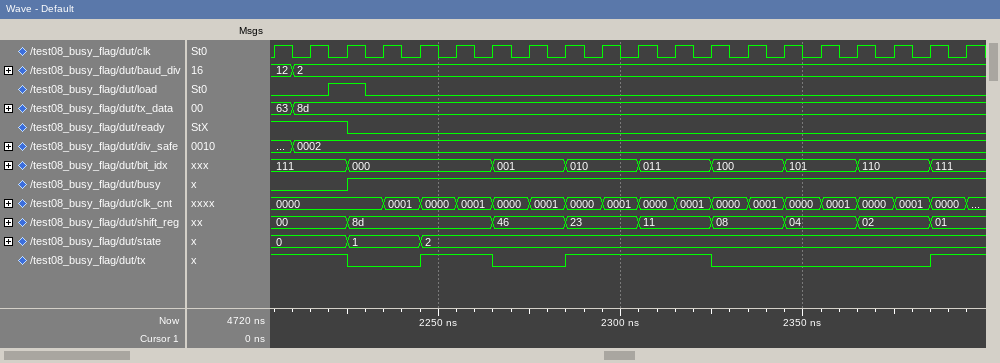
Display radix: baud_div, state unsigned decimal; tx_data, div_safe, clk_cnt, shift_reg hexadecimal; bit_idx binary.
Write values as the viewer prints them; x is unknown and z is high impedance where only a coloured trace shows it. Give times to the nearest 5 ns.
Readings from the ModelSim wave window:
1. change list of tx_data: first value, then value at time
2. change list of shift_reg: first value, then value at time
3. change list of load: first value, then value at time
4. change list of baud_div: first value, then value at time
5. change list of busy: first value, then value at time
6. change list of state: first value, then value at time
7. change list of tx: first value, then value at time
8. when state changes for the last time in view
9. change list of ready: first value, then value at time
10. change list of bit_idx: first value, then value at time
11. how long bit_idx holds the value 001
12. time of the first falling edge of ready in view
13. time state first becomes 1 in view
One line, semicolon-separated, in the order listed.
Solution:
63, 8d at 2210 ns; 00, 8d at 2225 ns, 46 at 2265 ns, 23 at 2285 ns, 11 at 2305 ns, 08 at 2325 ns, 04 at 2345 ns, 02 at 2365 ns, 01 at 2385 ns; 0, 1 at 2220 ns, 0 at 2230 ns; 12, 2 at 2210 ns; 0, 1 at 2225 ns; 0, 1 at 2225 ns, 2 at 2245 ns; 1, 0 at 2225 ns, 1 at 2245 ns, 0 at 2265 ns, 1 at 2285 ns, 0 at 2325 ns, 1 at 2385 ns; 2245 ns; 1, 0 at 2225 ns; 111, 000 at 2225 ns, 001 at 2265 ns, 010 at 2285 ns, 011 at 2305 ns, 100 at 2325 ns, 101 at 2345 ns, 110 at 2365 ns, 111 at 2385 ns; 20 ns; 2225 ns; 2225 ns
